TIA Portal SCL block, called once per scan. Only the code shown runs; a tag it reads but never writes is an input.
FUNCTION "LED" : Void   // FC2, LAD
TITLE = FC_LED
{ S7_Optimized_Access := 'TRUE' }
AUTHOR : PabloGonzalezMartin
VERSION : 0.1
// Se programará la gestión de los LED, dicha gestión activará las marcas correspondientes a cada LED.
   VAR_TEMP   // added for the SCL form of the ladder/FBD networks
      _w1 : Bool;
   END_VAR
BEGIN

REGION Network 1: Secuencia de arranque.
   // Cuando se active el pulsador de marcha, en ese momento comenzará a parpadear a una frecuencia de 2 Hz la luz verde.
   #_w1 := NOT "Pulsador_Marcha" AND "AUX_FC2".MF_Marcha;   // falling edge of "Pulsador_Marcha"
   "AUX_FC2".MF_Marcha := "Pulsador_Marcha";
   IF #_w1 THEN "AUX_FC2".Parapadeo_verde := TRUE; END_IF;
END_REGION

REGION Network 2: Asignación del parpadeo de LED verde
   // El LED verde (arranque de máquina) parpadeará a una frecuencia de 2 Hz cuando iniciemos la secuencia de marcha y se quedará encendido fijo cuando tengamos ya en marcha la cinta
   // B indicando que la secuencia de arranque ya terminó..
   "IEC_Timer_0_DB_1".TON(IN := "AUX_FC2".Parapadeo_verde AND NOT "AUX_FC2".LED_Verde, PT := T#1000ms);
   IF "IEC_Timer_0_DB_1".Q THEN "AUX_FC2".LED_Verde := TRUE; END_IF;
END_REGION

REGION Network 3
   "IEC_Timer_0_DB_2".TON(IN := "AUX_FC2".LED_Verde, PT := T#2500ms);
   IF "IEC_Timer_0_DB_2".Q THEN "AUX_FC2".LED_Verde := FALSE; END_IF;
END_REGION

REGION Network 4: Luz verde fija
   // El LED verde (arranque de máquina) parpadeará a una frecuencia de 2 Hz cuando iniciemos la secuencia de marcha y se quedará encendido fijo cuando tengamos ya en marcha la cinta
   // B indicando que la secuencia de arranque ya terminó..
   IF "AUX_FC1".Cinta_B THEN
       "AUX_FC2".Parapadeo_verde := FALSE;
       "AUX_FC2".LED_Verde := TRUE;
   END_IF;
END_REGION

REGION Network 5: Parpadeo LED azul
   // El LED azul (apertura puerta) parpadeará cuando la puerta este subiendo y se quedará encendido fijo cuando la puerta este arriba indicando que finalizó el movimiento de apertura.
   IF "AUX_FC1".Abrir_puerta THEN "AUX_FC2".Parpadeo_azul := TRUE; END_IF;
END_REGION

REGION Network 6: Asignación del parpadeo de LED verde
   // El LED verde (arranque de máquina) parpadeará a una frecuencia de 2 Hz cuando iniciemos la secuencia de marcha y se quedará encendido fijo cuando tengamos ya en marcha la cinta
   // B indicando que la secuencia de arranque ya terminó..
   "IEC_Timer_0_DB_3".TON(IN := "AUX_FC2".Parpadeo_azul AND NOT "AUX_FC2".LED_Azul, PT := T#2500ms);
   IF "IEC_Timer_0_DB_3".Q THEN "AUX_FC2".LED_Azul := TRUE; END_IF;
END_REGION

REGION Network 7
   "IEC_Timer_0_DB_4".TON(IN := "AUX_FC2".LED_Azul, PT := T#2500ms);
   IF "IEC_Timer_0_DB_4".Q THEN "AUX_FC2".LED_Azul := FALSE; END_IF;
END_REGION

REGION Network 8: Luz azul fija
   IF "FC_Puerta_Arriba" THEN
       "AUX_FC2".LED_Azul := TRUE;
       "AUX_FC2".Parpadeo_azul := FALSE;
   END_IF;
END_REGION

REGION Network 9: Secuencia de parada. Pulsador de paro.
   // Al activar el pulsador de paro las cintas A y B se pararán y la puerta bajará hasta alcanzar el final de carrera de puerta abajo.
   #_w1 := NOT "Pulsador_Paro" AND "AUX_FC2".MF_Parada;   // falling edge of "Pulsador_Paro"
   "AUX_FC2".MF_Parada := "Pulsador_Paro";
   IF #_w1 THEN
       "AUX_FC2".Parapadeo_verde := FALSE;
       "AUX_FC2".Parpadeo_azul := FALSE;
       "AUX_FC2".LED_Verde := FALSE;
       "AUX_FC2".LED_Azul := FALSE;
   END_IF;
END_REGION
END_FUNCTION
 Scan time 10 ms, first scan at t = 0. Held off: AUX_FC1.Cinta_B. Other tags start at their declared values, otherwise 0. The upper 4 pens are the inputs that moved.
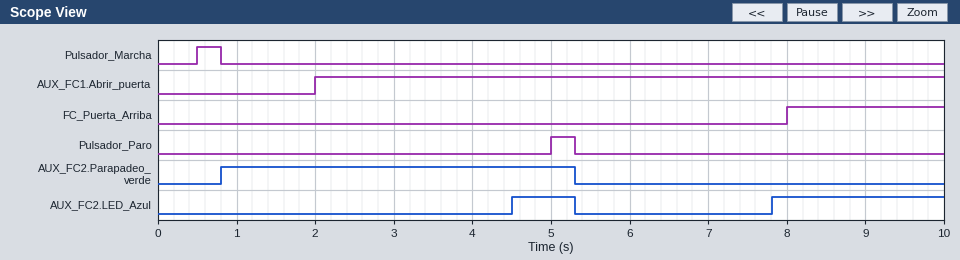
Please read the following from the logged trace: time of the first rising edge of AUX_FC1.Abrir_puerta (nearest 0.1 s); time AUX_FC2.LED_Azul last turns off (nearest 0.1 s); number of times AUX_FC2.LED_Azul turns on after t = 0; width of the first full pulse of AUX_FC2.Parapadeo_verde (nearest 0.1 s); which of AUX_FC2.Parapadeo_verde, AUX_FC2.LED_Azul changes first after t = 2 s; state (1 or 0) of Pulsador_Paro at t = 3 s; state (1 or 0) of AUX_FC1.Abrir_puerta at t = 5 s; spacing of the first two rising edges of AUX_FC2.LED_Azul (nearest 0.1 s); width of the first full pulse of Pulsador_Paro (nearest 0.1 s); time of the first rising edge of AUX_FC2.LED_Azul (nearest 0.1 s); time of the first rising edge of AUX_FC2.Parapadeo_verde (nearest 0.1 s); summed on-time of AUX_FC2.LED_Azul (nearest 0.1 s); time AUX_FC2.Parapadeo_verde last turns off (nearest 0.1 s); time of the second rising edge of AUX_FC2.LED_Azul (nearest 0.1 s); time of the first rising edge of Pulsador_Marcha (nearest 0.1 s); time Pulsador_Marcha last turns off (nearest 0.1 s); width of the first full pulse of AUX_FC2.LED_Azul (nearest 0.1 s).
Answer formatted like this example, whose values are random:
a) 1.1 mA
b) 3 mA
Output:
a) 2.0 s
b) 5.3 s
c) 2
d) 4.5 s
e) AUX_FC2.LED_Azul
f) 0
g) 1
h) 3.3 s
i) 0.3 s
j) 4.5 s
k) 0.8 s
l) 3.0 s
m) 5.3 s
n) 7.8 s
o) 0.5 s
p) 0.8 s
q) 0.8 s
